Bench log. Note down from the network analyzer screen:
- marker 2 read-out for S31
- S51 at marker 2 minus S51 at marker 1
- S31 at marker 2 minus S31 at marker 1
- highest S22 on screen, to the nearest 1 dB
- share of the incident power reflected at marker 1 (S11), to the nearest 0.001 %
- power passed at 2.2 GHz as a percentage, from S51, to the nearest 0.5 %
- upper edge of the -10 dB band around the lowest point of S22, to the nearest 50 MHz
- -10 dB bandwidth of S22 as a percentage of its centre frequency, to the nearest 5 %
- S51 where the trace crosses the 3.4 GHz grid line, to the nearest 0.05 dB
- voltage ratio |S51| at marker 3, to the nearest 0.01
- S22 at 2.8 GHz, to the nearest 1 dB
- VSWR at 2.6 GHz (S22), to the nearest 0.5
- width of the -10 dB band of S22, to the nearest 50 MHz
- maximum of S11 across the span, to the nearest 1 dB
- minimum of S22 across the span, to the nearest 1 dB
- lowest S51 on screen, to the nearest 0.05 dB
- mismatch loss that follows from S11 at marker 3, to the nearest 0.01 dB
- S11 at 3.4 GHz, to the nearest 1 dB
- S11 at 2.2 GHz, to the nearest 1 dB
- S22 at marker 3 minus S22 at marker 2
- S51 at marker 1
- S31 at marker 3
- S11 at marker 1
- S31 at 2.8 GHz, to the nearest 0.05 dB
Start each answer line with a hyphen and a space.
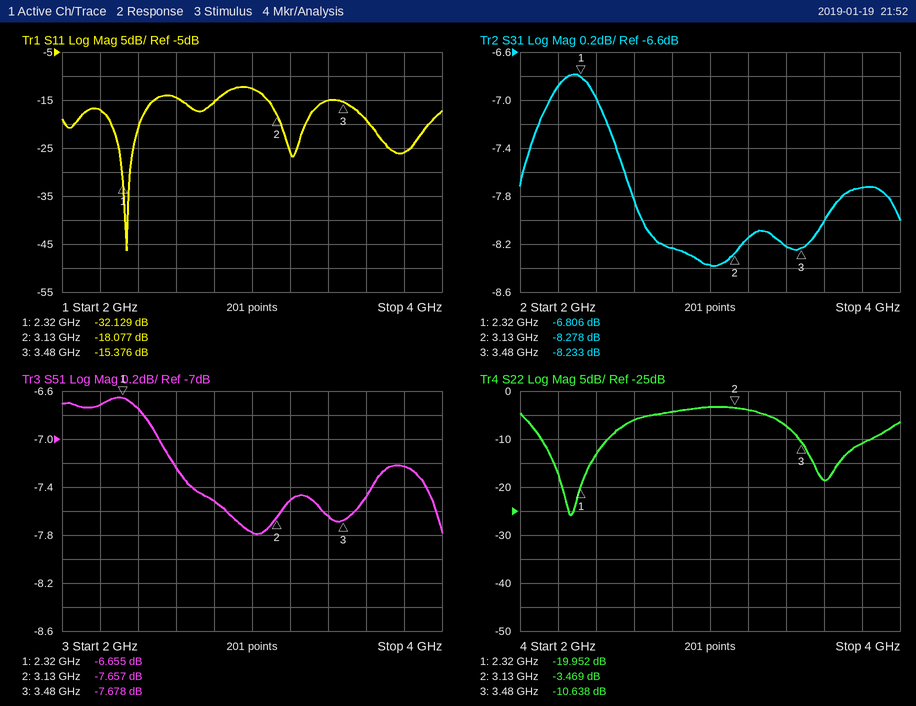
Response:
- -8.278 dB
- -1.002 dB
- -1.472 dB
- -3 dB
- 0.061 %
- 21.5 %
- 2.45 GHz
- 15 %
- -7.65 dB
- 0.41
- -4 dB
- 3.0
- 350 MHz
- -12 dB
- -26 dB
- -7.80 dB
- 0.13 dB
- -15 dB
- -17 dB
- -7.169 dB
- -6.655 dB
- -8.233 dB
- -32.129 dB
- -8.25 dB
